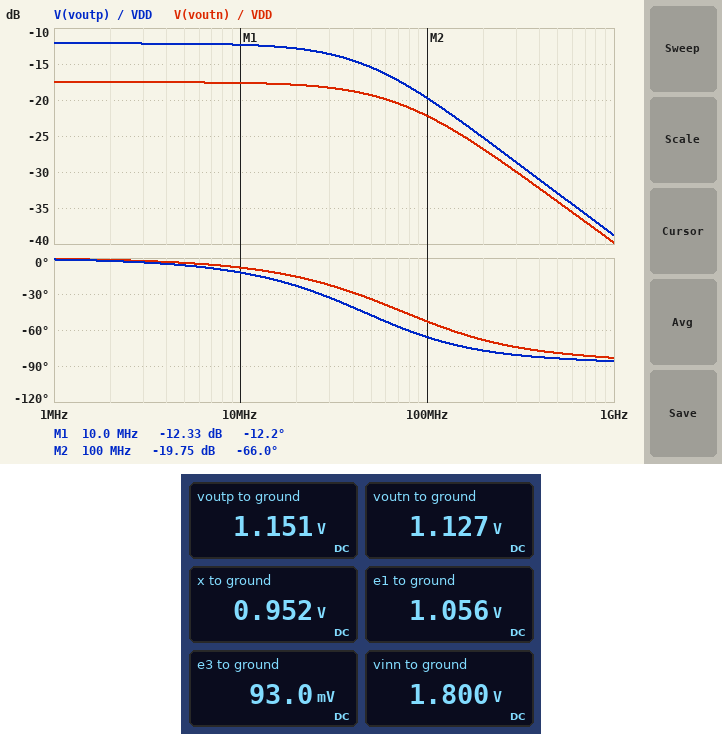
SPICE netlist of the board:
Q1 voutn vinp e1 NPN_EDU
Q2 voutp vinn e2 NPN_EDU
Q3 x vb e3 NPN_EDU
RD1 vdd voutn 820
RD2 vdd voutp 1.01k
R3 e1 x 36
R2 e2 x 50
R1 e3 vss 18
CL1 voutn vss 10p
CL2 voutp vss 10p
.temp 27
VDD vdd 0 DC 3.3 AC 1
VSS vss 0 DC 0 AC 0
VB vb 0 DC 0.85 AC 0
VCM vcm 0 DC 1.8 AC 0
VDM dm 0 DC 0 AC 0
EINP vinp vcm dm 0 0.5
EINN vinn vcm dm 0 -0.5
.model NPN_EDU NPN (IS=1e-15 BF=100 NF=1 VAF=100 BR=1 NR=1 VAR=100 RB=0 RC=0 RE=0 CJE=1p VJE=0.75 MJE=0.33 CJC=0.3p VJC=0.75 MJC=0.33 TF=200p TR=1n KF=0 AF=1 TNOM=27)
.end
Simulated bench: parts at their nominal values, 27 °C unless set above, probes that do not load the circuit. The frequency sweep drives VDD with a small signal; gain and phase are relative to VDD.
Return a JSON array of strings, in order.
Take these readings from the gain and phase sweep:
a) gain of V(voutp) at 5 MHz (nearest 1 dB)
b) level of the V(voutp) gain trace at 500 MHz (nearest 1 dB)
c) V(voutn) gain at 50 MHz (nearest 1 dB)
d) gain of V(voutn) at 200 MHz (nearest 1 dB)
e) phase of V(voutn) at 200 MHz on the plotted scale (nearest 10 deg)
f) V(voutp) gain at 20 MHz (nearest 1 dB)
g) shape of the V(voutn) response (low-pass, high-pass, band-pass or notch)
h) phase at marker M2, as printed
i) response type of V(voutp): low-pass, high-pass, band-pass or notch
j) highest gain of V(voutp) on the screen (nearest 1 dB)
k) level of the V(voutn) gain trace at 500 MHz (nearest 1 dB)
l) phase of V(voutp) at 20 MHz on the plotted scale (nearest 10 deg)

["-12 dB", "-33 dB", "-19 dB", "-27 dB", "-70 deg", "-13 dB", "low-pass", "-66.0 deg", "low-pass", "-12 dB", "-34 dB", "-20 deg"]
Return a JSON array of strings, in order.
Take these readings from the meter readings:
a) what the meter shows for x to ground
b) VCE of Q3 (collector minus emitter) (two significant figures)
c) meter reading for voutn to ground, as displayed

["0.952 V", "860 mV", "1.127 V"]
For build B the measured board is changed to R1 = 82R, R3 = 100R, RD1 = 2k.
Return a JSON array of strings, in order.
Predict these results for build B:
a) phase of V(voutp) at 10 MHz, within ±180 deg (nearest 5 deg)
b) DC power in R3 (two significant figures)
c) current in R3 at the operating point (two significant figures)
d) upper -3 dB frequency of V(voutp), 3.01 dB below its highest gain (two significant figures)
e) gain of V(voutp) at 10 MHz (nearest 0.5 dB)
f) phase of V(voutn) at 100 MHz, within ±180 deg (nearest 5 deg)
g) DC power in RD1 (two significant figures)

["-35 deg", "34 µW", "580 µA", "15 MHz", "-1.5 dB", "-85 deg", "660 µW"]
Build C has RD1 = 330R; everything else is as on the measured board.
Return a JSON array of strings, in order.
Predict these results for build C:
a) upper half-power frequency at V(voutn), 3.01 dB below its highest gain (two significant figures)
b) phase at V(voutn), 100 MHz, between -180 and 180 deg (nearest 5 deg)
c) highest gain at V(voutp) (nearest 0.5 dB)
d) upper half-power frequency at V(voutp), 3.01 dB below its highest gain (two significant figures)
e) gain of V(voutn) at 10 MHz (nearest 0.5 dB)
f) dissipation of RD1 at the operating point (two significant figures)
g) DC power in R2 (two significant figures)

["46 MHz", "-65 deg", "-11.5 dB", "45 MHz", "0 dB", "2.7 mW", "240 µW"]
